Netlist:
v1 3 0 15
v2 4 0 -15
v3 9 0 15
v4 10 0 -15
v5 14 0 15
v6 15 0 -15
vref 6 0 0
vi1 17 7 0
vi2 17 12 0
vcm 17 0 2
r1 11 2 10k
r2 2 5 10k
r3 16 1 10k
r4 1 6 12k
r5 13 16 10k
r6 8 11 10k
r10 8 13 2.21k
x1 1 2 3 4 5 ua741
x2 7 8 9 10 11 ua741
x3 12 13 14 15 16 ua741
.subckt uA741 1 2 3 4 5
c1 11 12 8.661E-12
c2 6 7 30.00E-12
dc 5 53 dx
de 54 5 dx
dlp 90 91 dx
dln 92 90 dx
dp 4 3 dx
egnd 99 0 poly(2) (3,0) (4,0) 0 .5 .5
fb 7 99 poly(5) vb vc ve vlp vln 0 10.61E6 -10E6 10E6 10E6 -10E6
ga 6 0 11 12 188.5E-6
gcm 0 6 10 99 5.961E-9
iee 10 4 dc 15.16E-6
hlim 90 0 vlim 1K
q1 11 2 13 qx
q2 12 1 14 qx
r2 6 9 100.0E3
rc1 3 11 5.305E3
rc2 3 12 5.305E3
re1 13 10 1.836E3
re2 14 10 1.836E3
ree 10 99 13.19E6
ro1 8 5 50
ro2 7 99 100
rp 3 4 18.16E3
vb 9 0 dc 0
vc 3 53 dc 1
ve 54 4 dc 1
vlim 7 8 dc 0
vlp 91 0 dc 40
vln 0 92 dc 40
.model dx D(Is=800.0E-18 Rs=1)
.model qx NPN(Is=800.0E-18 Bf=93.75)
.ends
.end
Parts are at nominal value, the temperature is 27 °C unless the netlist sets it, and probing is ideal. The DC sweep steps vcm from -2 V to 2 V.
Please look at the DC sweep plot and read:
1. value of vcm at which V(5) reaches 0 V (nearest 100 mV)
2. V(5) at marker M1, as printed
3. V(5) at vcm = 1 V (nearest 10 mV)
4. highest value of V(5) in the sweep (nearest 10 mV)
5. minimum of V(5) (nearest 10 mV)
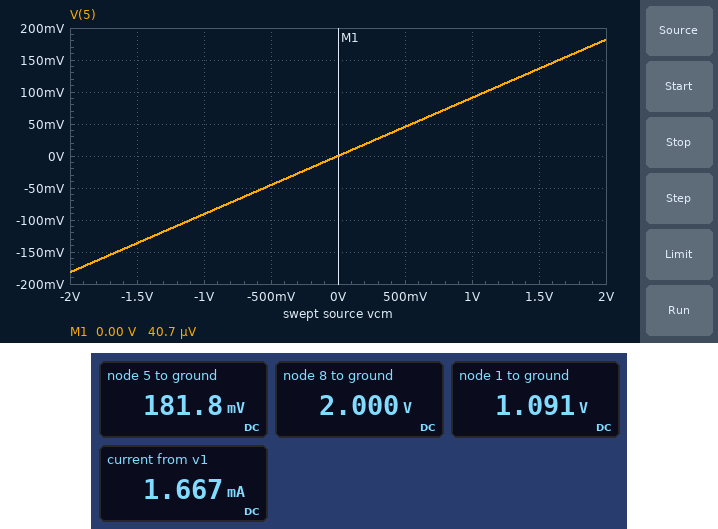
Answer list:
0 V
40.7 µV
90 mV
180 mV
-180 mV
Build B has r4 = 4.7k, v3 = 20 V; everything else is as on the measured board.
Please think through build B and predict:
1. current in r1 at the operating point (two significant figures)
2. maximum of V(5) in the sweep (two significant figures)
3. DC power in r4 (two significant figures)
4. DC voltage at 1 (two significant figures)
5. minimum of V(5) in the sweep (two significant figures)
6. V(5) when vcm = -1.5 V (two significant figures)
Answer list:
140 µA
720 mV
87 µW
640 mV
-720 mV
540 mV
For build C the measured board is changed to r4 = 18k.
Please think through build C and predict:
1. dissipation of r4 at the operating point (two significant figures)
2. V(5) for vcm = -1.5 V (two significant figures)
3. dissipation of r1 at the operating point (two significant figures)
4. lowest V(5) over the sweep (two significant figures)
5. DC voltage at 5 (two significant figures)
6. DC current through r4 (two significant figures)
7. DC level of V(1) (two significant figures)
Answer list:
92 µW
-430 mV
51 µW
-570 mV
570 mV
71 µA
1.3 V
